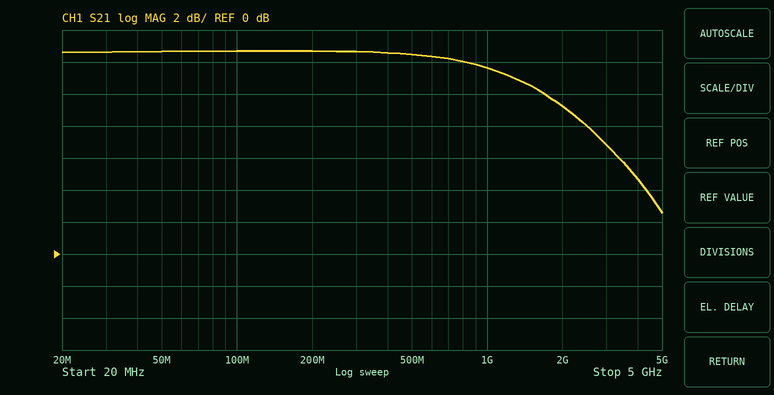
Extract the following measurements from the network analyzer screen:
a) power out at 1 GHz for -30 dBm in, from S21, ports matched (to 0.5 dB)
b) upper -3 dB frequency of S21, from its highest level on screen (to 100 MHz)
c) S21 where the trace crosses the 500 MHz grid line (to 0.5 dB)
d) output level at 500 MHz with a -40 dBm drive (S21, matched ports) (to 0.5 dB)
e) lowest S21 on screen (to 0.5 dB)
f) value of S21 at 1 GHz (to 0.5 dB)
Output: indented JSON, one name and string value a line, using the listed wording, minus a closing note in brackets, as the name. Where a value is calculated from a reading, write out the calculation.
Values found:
{
  "power out at 1 GHz for -30 dBm in, from S21, ports matched": "-30 dBm + (11.5 dB) = -18.5 dBm",
  "upper -3 dB frequency of S21, from its highest level on screen": "1.8 GHz",
  "S21 where the trace crosses the 500 MHz grid line": "12.5 dB",
  "output level at 500 MHz with a -40 dBm drive (S21, matched ports)": "-40 dBm + (12.5 dB) = -27.5 dBm",
  "lowest S21 on screen": "2.5 dB",
  "value of S21 at 1 GHz": "11.5 dB"
}
